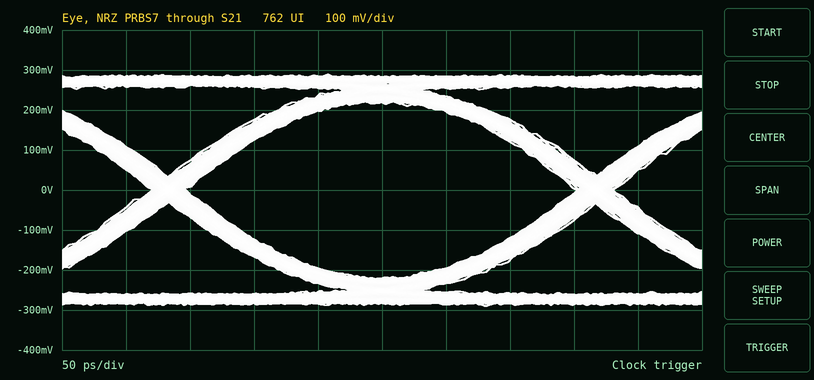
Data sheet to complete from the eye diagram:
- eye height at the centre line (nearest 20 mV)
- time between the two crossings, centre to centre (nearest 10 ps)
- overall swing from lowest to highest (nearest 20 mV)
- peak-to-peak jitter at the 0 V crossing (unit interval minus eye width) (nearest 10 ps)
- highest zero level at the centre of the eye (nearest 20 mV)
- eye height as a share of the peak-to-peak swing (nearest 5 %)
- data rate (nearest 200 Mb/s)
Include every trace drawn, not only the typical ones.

440 mV
330 ps
580 mV
30 ps
-220 mV
75 %
3.0 Gb/s
